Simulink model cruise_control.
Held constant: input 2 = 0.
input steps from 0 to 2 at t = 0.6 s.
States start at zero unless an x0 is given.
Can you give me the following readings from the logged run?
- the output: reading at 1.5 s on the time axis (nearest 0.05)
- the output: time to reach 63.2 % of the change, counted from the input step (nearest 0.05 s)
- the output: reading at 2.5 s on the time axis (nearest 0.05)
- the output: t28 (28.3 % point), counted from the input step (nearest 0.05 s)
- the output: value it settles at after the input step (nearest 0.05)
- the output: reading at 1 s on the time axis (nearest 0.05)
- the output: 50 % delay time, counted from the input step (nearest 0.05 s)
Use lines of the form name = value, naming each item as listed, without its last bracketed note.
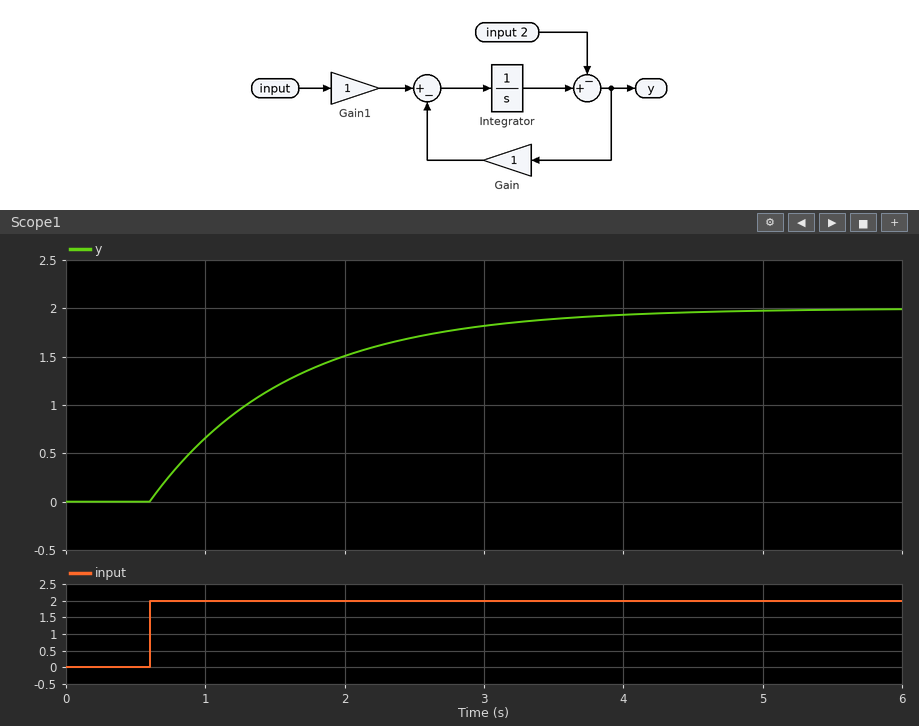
the output: reading at 1.5 s on the time axis = 1.20
the output: time to reach 63.2 % of the change, counted from the input step = 1.00 s
the output: reading at 2.5 s on the time axis = 1.70
the output: t28 (28.3 % point), counted from the input step = 0.35 s
the output: value it settles at after the input step = 2.00
the output: reading at 1 s on the time axis = 0.65
the output: 50 % delay time, counted from the input step = 0.70 s
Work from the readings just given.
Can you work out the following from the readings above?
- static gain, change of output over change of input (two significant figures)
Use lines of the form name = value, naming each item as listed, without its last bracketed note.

static gain, change of output over change of input = 1.0
